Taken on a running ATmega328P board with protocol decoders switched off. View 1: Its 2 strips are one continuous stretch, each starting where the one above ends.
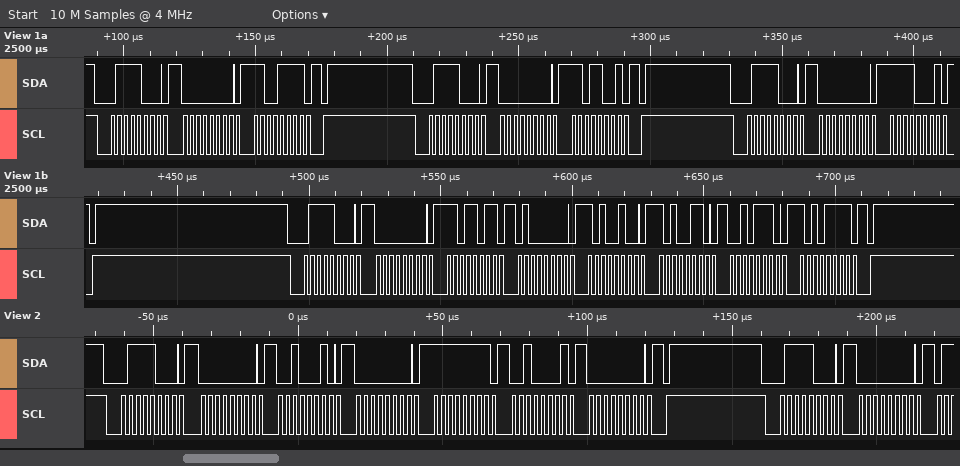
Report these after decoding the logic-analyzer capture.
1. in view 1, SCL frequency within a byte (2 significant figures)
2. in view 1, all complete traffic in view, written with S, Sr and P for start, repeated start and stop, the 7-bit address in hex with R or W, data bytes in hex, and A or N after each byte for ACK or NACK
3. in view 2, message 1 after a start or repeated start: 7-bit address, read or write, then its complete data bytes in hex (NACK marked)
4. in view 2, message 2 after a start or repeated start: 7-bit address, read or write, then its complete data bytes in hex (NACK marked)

400 kHz
S 3CW A 00 A CF A P S 3CW A 00 A D9 A P S 3CW A 00 A F1 A P S 3CW A 00 A DB A 40 A A4 A A6 A 2E A AF A P
0x3C write: 00 22 00 FF 21 00
0x3C write: 00
